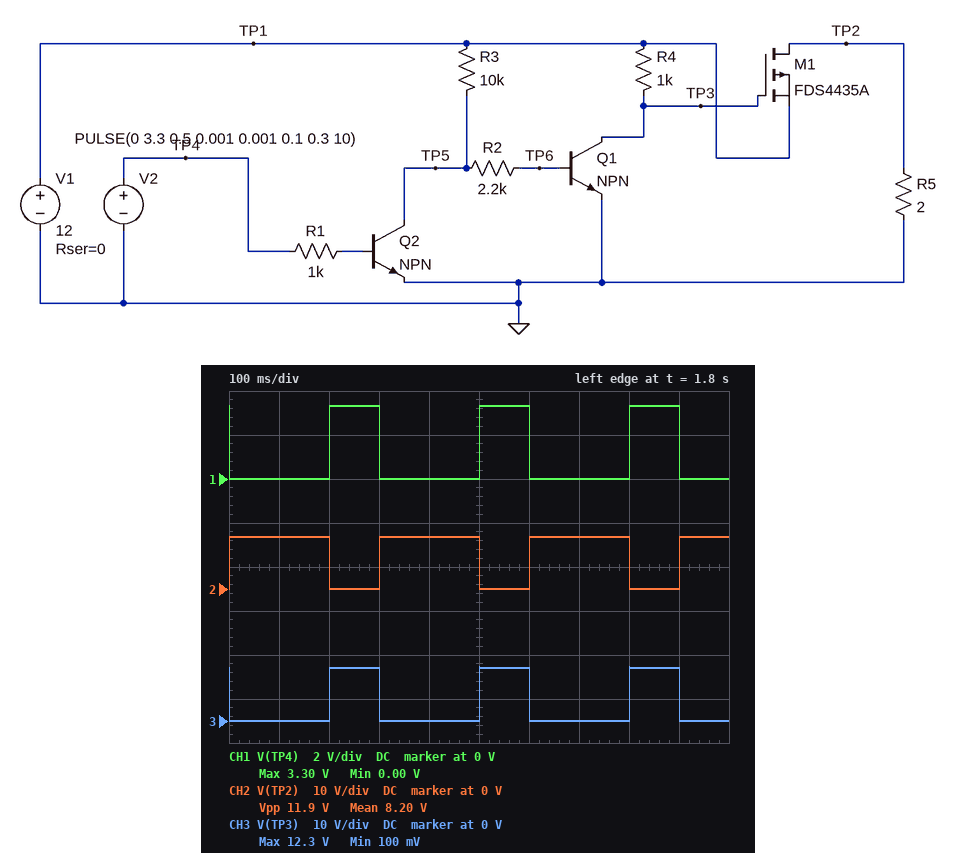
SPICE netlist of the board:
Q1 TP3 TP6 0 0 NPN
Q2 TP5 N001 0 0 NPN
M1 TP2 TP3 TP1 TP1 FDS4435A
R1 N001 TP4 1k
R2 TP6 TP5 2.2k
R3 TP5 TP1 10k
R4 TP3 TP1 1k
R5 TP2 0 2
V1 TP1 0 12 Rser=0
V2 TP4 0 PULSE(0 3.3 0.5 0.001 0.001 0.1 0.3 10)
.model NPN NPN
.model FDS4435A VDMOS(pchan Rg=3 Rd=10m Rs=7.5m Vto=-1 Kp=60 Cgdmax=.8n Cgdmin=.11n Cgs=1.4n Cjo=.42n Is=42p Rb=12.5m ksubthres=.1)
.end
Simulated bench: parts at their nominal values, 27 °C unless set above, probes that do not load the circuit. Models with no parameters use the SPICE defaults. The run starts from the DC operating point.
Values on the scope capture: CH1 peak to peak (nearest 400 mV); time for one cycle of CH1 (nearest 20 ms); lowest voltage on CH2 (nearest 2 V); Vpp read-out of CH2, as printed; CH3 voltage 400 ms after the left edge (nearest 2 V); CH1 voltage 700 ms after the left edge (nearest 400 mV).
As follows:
3.2 V
300 ms
0 V
11.9 V
0 V
0 V
